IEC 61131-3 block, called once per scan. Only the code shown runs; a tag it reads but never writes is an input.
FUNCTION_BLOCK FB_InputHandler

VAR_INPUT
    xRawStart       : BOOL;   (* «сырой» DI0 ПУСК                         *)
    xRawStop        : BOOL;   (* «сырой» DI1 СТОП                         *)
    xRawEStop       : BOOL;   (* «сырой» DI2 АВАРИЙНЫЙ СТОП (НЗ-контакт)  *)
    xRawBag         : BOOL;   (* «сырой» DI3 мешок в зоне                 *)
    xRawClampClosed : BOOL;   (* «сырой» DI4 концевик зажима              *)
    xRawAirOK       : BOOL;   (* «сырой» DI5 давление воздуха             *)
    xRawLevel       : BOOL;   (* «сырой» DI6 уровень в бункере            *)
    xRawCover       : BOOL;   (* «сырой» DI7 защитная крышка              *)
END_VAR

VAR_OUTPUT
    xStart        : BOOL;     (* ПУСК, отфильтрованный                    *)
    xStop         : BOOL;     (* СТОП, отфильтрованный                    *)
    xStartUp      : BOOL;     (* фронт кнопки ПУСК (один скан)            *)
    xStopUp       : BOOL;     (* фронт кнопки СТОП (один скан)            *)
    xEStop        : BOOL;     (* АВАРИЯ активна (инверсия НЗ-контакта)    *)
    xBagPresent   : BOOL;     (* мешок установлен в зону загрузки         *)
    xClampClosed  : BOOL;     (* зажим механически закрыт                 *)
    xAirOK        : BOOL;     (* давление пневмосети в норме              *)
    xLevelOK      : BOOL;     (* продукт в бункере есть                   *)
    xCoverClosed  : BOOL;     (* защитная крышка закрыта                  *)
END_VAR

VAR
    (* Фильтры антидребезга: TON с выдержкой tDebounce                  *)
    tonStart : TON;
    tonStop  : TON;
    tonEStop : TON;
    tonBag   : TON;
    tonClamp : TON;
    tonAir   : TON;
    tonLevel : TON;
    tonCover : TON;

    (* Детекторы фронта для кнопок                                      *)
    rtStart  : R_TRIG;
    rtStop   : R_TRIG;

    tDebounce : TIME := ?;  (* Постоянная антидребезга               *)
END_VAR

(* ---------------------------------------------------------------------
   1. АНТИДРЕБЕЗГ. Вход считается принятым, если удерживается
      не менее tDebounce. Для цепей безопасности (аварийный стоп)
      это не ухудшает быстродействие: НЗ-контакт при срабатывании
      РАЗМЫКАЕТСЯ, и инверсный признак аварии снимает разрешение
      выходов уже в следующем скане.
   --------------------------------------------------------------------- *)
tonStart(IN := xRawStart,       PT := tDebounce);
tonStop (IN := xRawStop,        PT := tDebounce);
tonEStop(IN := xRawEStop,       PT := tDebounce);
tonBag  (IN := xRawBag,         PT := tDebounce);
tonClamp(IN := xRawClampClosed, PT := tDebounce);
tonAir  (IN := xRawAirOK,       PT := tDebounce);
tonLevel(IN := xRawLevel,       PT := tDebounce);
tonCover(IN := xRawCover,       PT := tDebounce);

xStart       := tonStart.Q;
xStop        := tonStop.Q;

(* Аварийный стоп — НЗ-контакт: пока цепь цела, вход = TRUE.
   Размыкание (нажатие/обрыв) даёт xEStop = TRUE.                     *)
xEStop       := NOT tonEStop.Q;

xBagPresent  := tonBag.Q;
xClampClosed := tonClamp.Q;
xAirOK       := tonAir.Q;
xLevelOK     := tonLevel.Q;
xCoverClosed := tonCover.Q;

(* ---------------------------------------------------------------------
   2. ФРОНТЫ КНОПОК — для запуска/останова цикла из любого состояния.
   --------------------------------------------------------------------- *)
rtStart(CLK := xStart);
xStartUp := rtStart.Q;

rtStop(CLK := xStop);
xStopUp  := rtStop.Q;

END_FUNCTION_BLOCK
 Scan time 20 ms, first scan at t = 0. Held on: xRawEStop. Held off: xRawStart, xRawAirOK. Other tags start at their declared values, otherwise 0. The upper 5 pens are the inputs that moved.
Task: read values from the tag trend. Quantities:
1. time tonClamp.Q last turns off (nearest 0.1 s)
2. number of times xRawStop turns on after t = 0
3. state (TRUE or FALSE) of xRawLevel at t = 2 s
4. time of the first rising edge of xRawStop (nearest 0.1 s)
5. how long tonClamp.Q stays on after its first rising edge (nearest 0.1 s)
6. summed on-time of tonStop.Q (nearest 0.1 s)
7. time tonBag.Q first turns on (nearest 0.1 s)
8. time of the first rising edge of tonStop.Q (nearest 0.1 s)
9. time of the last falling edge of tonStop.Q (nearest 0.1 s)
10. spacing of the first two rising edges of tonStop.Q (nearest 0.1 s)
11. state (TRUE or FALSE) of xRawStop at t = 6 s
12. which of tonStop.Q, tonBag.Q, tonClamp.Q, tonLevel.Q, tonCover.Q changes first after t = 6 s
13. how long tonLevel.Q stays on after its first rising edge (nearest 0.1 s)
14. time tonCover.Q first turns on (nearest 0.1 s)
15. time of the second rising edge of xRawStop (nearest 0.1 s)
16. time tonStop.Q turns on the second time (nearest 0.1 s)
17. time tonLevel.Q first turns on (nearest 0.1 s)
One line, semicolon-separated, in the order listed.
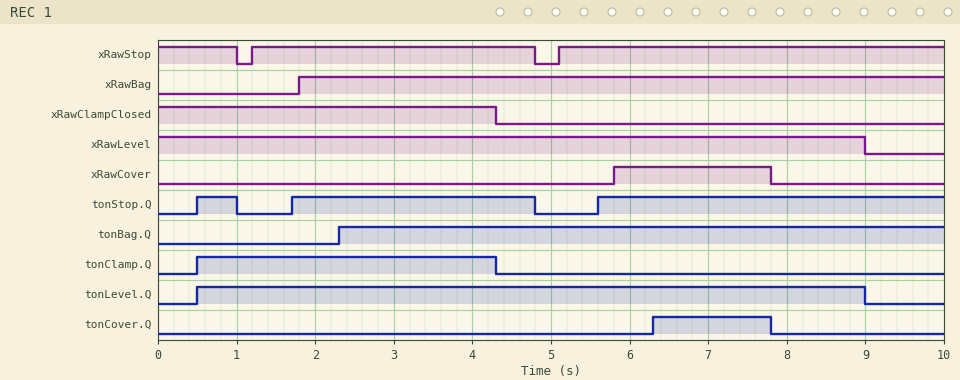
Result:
4.3 s; 2; TRUE; 1.2 s; 3.8 s; 8.0 s; 2.3 s; 0.5 s; 4.8 s; 1.2 s; TRUE; tonCover.Q; 8.5 s; 6.3 s; 5.1 s; 1.7 s; 0.5 s
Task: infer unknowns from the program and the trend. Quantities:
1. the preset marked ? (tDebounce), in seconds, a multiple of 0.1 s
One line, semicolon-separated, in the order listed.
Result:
0.5 s
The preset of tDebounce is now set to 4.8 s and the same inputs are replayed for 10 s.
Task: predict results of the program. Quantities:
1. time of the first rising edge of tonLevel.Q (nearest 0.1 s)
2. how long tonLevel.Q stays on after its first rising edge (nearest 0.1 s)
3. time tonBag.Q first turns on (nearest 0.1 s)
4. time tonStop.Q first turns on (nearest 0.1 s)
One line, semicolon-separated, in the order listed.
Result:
4.8 s; 4.2 s; 6.6 s; 9.9 s
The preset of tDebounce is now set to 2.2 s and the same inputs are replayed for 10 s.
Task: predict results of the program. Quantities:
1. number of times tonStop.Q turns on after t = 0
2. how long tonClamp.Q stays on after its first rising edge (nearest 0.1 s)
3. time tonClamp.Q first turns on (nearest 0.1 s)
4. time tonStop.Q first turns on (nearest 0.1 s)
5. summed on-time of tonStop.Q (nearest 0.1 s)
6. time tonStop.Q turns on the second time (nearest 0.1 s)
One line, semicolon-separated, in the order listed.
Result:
2; 2.1 s; 2.2 s; 3.4 s; 4.1 s; 7.3 s
